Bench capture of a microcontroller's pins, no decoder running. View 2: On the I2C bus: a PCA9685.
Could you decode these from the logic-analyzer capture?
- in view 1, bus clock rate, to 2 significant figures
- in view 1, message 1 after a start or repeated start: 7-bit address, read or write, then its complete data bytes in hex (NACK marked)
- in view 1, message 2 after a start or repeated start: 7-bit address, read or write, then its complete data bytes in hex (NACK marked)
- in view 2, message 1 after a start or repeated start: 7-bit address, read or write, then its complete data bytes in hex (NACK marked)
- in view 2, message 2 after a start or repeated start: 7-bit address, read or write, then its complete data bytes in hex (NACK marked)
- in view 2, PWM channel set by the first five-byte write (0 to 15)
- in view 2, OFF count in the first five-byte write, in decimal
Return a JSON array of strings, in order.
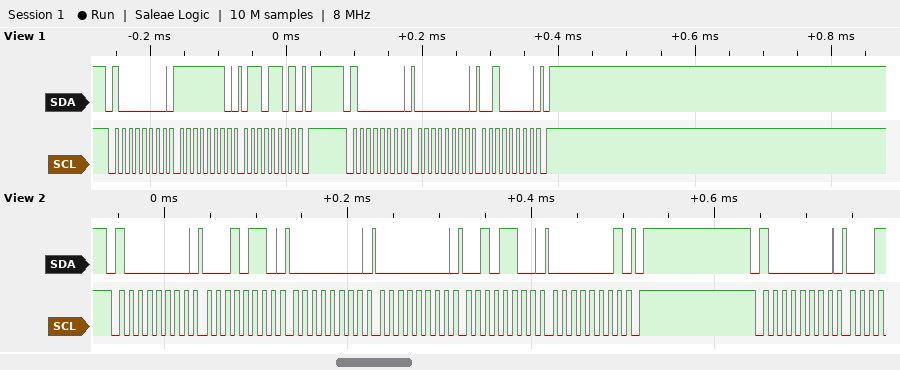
["100 kHz", "0x40 write: FE 6D", "0x40 write: 00 20", "0x40 write: 16 00 00 2C 01", "0x40 write", "4", "300"]
